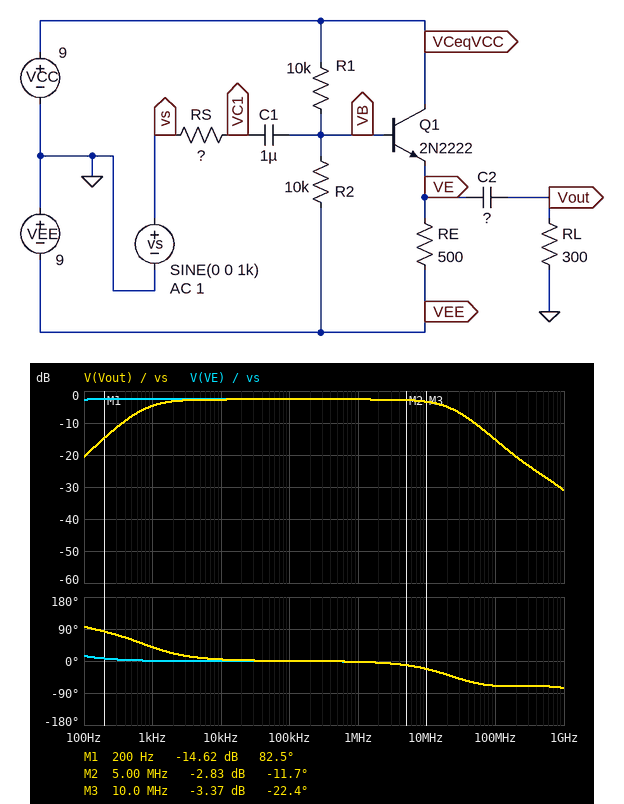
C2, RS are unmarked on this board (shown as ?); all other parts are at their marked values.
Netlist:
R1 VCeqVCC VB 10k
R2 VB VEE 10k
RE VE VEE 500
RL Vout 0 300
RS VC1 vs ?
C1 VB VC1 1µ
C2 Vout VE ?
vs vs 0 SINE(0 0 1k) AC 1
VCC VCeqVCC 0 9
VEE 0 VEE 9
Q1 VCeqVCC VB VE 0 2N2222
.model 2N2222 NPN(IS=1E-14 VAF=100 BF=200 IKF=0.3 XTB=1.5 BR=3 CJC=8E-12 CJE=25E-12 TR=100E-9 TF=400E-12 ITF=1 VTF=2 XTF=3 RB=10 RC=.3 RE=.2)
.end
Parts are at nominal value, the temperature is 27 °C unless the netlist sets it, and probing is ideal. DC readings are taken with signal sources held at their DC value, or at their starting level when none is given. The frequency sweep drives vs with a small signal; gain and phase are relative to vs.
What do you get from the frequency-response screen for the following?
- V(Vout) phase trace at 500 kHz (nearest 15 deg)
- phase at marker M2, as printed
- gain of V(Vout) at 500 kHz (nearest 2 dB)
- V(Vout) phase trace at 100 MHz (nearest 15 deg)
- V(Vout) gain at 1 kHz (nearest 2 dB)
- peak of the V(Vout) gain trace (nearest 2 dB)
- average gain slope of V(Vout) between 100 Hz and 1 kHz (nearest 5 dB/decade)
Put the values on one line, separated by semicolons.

0 deg; -11.7 deg; -2 dB; -75 deg; -4 dB; -2 dB; 15 dB/decade
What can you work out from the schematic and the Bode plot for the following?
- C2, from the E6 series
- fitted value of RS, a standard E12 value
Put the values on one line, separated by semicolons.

680 nF; 1.5 kΩ
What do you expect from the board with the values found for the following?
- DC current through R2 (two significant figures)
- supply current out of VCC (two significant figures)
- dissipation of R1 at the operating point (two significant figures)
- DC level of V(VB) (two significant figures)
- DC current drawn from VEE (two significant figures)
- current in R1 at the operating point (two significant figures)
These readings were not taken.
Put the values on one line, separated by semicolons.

860 µA; 17 mA; 8.8 mW; -380 mV; 17 mA; 940 µA
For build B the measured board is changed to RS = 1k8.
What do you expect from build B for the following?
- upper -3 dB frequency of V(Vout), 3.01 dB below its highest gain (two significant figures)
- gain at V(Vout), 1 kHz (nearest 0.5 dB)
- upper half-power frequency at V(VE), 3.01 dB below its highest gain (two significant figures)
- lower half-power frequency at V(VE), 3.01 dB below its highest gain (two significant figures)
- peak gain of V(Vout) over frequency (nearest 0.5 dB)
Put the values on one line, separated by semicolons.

21 MHz; -5.0 dB; 20 MHz; 24 Hz; -3.0 dB
